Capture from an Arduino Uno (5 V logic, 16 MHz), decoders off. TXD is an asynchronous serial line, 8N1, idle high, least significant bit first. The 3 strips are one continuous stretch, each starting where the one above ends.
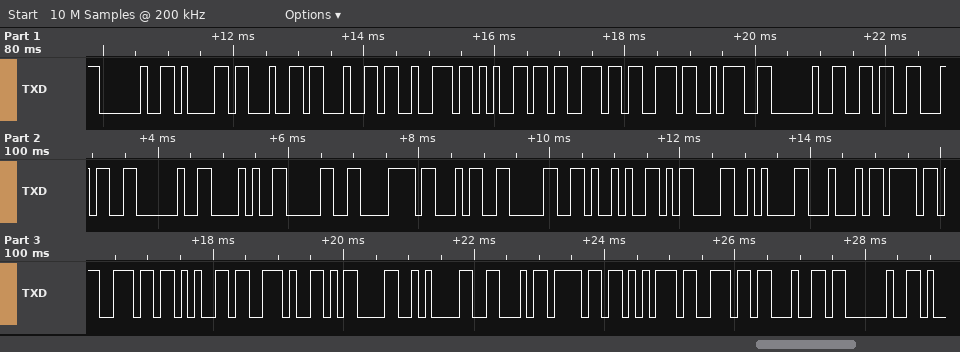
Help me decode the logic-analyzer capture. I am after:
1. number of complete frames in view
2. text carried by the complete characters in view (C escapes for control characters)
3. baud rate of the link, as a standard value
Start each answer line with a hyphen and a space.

- 34
- " address: 64 (0x40)\r\nDone.\r\nFound "
- 9600 baud
